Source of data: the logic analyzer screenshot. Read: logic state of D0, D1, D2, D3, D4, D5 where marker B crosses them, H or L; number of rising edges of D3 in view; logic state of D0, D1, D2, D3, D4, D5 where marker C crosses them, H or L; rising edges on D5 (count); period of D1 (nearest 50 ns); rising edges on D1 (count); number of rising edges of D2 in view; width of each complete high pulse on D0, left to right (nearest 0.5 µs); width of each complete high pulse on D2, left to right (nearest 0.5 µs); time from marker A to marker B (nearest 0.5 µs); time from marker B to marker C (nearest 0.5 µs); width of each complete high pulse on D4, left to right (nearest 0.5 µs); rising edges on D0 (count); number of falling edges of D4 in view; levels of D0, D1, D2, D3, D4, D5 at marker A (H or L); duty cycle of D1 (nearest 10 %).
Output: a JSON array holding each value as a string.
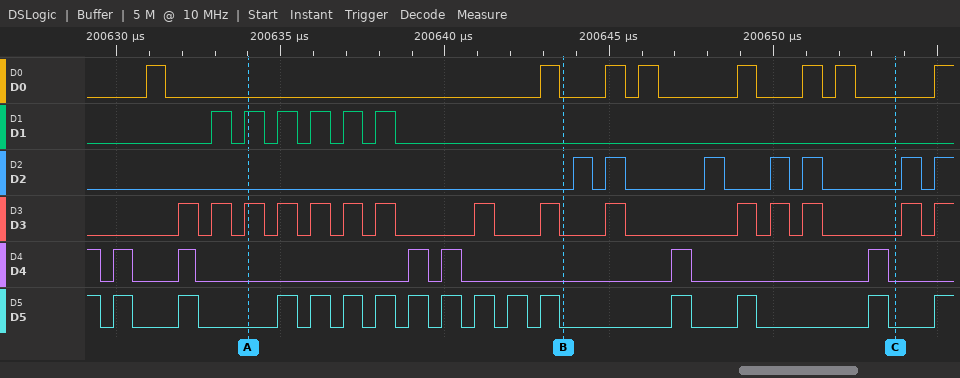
["D0=L, D1=L, D2=L, D3=L, D4=L, D5=L", "15", "D0=L, D1=L, D2=L, D3=L, D4=L, D5=L", "15", "1000 ns", "6", "7", "0.5 µs, 0.5 µs, 0.5 µs, 0.5 µs, 0.5 µs, 0.5 µs, 0.5 µs", "0.5 µs, 0.5 µs, 0.5 µs, 0.5 µs, 0.5 µs, 0.5 µs", "9.5 µs", "10 µs", "0.5 µs, 0.5 µs, 0.5 µs, 0.5 µs, 0.5 µs, 0.5 µs", "8", "7", "D0=L, D1=H, D2=L, D3=H, D4=L, D5=L", "60 %"]
